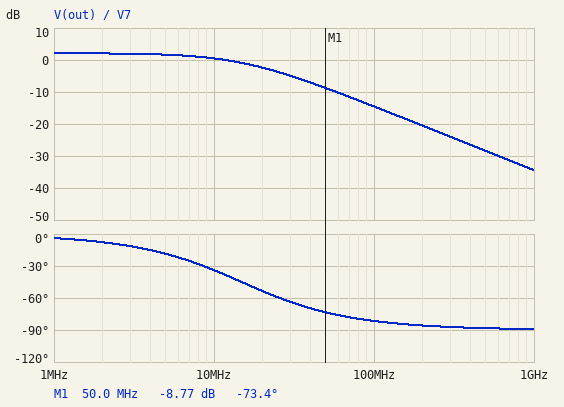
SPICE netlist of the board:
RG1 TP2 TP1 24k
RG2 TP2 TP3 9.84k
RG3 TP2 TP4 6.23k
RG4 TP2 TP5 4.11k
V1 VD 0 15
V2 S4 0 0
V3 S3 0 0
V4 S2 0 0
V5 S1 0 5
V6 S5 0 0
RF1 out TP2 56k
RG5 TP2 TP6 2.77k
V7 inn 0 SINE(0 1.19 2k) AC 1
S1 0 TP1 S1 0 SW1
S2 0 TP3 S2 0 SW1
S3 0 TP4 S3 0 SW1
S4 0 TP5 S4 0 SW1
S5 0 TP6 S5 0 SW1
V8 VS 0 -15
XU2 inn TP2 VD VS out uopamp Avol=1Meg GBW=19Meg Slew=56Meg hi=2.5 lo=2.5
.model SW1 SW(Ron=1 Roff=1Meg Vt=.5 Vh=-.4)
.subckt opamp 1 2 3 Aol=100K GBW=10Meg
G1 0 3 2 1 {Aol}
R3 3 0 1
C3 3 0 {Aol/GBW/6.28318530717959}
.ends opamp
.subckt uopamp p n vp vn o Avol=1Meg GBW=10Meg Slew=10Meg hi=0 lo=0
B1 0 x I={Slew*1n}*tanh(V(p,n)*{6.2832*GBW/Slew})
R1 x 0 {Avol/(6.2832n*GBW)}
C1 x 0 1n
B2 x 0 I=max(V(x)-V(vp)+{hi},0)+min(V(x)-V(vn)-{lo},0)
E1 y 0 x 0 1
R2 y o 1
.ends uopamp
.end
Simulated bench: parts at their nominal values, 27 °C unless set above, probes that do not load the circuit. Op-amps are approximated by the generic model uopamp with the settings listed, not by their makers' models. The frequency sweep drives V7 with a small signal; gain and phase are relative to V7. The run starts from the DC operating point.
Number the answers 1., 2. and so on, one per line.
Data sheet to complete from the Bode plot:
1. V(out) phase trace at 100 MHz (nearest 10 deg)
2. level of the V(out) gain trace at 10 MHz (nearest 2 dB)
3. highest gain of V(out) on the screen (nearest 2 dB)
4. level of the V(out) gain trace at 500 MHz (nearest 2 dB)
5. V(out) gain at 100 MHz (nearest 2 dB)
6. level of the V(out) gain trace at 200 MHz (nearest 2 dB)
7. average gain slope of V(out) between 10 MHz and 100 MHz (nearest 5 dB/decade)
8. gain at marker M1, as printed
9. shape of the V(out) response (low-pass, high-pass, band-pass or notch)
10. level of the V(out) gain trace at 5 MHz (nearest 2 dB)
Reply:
1. -80 deg
2. 0 dB
3. 2 dB
4. -28 dB
5. -14 dB
6. -20 dB
7. -15 dB/decade
8. -8.77 dB
9. low-pass
10. 2 dB
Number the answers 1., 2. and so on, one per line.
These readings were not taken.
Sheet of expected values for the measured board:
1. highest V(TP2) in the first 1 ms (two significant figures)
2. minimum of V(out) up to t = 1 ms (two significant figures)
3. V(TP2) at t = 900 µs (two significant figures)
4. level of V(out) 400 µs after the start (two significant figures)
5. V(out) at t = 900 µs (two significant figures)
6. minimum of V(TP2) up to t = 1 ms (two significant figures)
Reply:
1. 1.2 V
2. -4.2 V
3. -1.1 V
4. -4.0 V
5. -4.0 V
6. -1.2 V
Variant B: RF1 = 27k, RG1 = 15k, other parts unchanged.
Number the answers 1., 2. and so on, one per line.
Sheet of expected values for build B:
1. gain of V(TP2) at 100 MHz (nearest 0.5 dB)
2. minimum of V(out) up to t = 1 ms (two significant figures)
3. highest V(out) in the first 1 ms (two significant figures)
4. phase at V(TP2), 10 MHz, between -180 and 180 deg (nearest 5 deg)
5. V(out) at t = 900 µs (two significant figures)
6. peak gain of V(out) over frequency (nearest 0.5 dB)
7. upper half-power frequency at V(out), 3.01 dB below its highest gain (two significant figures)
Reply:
1. -15.5 dB
2. -3.5 V
3. 3.5 V
4. -30 deg
5. -3.3 V
6. 1.0 dB
7. 17 MHz
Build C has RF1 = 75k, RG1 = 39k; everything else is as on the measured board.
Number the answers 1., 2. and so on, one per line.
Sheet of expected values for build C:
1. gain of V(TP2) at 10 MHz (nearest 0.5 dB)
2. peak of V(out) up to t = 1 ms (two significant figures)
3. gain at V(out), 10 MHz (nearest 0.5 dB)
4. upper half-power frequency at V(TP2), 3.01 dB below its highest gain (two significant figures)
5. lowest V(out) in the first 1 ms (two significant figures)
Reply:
1. -2.0 dB
2. 3.8 V
3. 1.0 dB
4. 14 MHz
5. -3.8 V
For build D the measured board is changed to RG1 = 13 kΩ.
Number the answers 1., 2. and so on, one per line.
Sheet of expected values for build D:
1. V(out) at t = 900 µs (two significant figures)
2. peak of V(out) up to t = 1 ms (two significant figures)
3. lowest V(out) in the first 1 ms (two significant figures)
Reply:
1. -6.3 V
2. 6.6 V
3. -6.6 V
